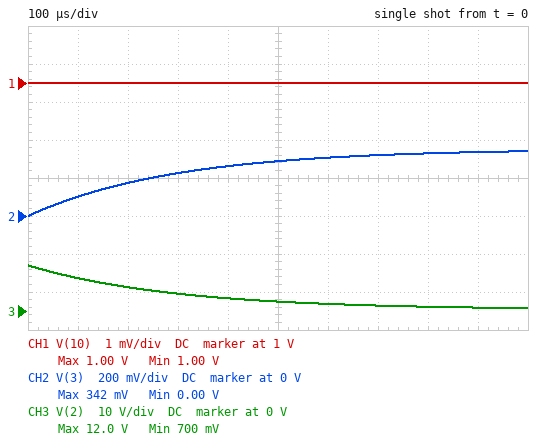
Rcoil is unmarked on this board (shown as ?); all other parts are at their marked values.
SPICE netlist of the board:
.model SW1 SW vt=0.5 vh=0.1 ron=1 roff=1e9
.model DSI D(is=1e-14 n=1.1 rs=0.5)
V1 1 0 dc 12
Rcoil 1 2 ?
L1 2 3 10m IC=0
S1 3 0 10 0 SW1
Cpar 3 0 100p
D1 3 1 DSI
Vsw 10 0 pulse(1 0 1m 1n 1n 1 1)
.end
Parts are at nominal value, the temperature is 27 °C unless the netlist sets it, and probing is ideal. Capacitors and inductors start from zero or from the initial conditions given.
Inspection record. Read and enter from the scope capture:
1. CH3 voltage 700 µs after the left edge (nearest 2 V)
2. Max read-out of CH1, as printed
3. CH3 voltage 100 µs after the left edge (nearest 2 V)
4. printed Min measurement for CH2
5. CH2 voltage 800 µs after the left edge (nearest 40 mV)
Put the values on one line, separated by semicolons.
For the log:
2 V; 1.00 V; 8 V; 0.00 V; 320 mV
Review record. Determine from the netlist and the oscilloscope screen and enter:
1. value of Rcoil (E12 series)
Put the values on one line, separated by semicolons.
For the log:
33 Ω
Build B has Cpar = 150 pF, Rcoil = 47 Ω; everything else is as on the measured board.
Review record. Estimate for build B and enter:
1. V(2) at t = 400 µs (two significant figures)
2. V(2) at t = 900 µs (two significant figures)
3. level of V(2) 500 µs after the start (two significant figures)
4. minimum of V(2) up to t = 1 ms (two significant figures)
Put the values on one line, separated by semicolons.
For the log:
2.0 V; 410 mV; 1.3 V; 350 mV
